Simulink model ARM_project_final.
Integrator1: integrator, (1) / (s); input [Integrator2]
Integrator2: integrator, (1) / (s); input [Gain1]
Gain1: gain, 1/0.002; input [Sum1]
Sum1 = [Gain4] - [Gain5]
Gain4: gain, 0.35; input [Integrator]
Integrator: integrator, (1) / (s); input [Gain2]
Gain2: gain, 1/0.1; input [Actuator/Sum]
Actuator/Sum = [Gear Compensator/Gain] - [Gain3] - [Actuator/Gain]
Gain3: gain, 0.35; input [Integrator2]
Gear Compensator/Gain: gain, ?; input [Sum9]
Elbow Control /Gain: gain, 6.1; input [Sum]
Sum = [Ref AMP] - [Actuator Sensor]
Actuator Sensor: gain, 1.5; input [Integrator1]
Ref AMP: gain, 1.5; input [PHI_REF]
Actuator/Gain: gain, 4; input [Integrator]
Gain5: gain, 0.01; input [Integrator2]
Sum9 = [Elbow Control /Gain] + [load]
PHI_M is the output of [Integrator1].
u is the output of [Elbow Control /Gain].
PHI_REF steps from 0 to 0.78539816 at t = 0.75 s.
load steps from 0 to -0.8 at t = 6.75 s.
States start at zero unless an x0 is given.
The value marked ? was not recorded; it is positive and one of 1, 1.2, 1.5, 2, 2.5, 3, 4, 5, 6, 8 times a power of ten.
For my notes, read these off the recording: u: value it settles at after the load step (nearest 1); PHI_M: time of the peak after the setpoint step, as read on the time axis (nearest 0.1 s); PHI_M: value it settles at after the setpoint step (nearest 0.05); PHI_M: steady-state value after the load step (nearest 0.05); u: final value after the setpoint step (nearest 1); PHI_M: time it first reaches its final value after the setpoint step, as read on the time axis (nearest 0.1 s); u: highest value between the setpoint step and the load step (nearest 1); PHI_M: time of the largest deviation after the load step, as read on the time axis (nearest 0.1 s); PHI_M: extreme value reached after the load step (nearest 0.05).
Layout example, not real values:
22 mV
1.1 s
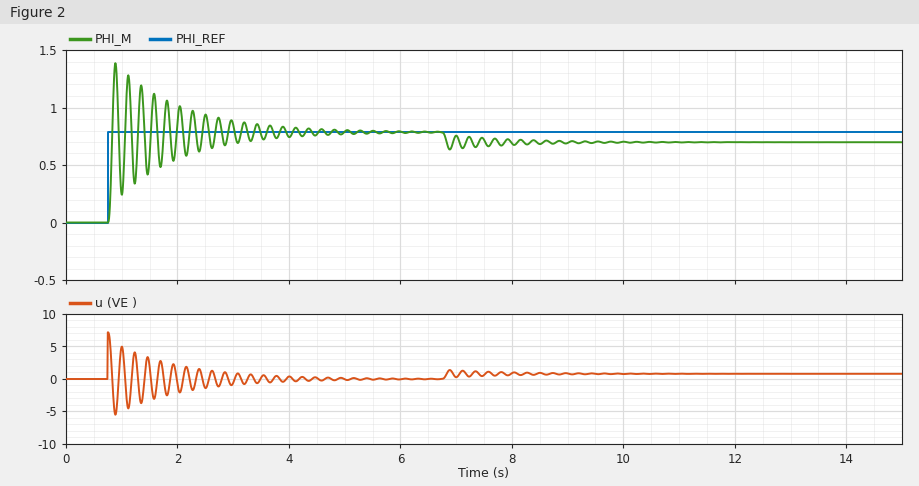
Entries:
1
0.9 s
0.80
0.70
0
0.8 s
7
6.9 s
0.65
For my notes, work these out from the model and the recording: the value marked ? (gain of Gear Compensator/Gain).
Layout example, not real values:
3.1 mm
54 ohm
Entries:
2
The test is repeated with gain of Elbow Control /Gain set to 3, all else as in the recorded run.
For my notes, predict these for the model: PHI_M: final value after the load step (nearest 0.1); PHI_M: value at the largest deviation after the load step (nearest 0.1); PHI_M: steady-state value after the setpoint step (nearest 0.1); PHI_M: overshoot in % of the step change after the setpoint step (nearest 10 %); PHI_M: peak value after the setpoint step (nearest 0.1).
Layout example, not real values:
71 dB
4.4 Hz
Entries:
0.6
0.5
0.8
40 %
1.1
